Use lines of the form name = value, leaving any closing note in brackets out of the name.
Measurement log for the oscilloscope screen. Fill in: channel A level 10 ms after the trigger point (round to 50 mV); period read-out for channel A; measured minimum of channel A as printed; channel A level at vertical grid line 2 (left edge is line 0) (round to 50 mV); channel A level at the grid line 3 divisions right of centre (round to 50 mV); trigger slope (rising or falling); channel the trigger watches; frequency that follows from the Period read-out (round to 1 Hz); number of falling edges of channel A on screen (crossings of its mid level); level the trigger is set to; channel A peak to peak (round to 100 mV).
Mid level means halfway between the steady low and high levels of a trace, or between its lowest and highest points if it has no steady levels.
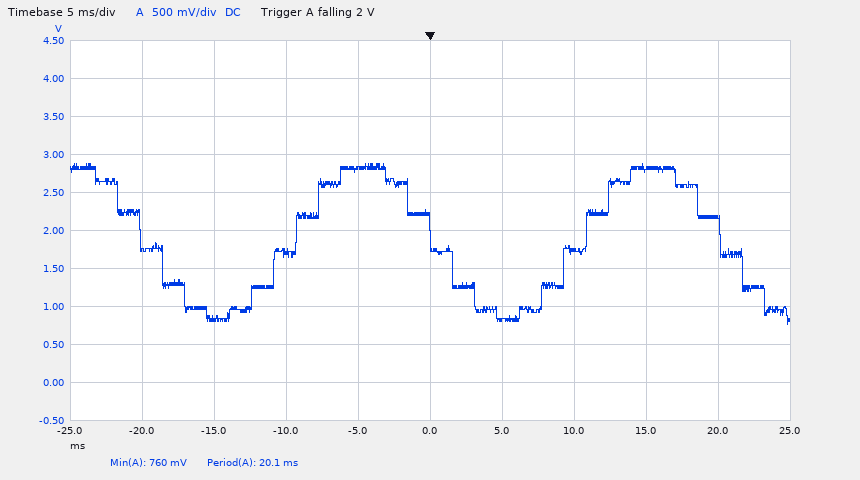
channel A level 10 ms after the trigger point = 1.75 V
period read-out for channel A = 20.1 ms
measured minimum of channel A as printed = 760 mV
channel A level at vertical grid line 2 (left edge is line 0) = 850 mV
channel A level at the grid line 3 divisions right of centre = 2.80 V
trigger slope = falling
channel the trigger watches = channel A
frequency that follows from the Period read-out = 50 Hz
number of falling edges of channel A on screen = 3
level the trigger is set to = 2 V
channel A peak to peak = 2.10 V
